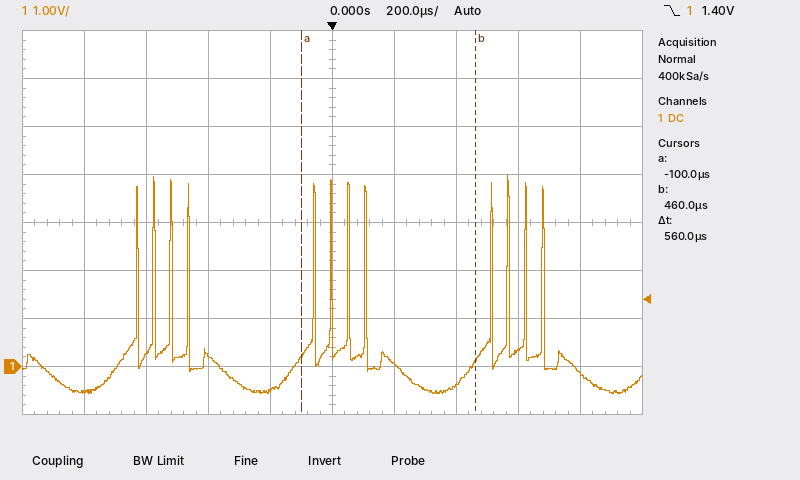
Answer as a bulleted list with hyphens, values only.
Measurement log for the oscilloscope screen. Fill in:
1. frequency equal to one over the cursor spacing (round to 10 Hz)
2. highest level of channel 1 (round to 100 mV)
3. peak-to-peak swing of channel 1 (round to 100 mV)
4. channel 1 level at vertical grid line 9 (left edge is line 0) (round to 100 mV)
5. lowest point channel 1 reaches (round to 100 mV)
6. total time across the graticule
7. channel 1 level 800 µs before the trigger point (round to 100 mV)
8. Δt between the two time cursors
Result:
- 1.79 kHz
- 4.0 V
- 4.6 V
- -100 mV
- -600 mV
- 2 ms
- -500 mV
- 560 µs
